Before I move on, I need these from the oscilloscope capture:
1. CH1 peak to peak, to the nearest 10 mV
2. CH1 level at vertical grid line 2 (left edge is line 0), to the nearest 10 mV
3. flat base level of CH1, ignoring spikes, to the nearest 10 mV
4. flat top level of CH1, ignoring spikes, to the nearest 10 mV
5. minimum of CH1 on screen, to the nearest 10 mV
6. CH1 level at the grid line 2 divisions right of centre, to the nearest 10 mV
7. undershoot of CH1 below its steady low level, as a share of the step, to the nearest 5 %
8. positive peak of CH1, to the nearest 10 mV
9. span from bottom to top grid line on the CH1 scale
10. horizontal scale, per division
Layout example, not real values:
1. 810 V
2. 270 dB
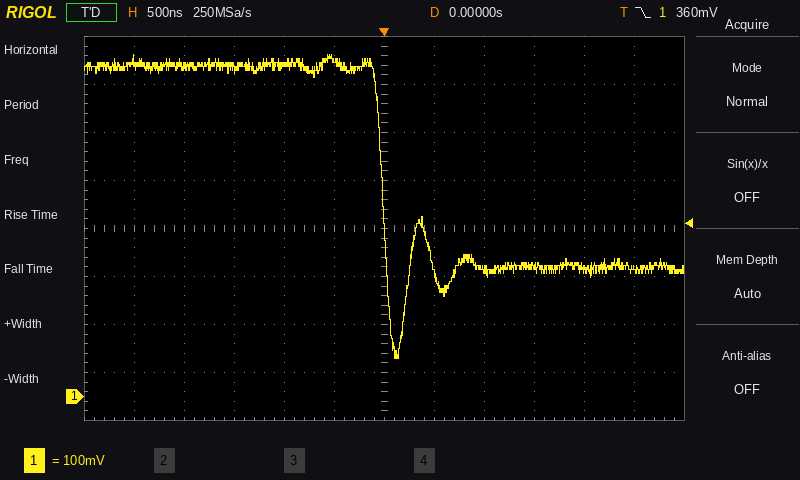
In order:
1. 630 mV
2. 690 mV
3. 270 mV
4. 690 mV
5. 80 mV
6. 260 mV
7. 45 %
8. 710 mV
9. 800 mV
10. 500 ns
